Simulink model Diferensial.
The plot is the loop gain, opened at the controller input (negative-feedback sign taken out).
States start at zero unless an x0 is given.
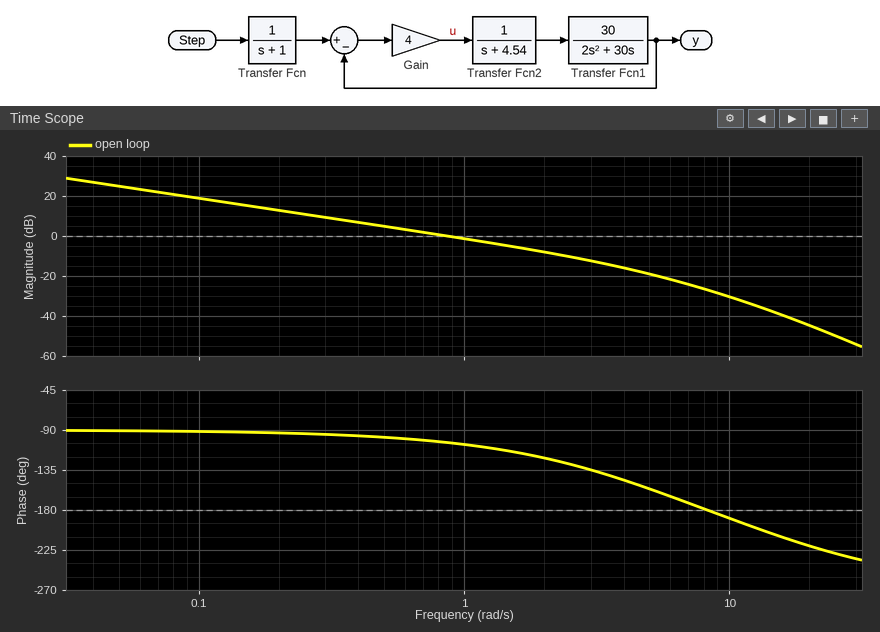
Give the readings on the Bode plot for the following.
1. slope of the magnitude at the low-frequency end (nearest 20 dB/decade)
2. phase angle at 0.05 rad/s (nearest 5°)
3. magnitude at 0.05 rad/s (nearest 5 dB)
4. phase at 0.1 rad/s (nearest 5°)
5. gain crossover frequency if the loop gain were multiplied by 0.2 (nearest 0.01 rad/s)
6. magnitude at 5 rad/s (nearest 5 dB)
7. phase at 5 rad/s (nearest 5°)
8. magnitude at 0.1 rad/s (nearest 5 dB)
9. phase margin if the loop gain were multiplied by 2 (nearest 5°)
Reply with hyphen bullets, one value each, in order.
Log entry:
- -20 dB/decade
- -90°
- 25 dB
- -90°
- 0.18 rad/s
- -20 dB
- -155°
- 20 dB
- 65°
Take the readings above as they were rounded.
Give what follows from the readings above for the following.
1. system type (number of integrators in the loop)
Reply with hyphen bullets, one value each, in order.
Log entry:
- 1
